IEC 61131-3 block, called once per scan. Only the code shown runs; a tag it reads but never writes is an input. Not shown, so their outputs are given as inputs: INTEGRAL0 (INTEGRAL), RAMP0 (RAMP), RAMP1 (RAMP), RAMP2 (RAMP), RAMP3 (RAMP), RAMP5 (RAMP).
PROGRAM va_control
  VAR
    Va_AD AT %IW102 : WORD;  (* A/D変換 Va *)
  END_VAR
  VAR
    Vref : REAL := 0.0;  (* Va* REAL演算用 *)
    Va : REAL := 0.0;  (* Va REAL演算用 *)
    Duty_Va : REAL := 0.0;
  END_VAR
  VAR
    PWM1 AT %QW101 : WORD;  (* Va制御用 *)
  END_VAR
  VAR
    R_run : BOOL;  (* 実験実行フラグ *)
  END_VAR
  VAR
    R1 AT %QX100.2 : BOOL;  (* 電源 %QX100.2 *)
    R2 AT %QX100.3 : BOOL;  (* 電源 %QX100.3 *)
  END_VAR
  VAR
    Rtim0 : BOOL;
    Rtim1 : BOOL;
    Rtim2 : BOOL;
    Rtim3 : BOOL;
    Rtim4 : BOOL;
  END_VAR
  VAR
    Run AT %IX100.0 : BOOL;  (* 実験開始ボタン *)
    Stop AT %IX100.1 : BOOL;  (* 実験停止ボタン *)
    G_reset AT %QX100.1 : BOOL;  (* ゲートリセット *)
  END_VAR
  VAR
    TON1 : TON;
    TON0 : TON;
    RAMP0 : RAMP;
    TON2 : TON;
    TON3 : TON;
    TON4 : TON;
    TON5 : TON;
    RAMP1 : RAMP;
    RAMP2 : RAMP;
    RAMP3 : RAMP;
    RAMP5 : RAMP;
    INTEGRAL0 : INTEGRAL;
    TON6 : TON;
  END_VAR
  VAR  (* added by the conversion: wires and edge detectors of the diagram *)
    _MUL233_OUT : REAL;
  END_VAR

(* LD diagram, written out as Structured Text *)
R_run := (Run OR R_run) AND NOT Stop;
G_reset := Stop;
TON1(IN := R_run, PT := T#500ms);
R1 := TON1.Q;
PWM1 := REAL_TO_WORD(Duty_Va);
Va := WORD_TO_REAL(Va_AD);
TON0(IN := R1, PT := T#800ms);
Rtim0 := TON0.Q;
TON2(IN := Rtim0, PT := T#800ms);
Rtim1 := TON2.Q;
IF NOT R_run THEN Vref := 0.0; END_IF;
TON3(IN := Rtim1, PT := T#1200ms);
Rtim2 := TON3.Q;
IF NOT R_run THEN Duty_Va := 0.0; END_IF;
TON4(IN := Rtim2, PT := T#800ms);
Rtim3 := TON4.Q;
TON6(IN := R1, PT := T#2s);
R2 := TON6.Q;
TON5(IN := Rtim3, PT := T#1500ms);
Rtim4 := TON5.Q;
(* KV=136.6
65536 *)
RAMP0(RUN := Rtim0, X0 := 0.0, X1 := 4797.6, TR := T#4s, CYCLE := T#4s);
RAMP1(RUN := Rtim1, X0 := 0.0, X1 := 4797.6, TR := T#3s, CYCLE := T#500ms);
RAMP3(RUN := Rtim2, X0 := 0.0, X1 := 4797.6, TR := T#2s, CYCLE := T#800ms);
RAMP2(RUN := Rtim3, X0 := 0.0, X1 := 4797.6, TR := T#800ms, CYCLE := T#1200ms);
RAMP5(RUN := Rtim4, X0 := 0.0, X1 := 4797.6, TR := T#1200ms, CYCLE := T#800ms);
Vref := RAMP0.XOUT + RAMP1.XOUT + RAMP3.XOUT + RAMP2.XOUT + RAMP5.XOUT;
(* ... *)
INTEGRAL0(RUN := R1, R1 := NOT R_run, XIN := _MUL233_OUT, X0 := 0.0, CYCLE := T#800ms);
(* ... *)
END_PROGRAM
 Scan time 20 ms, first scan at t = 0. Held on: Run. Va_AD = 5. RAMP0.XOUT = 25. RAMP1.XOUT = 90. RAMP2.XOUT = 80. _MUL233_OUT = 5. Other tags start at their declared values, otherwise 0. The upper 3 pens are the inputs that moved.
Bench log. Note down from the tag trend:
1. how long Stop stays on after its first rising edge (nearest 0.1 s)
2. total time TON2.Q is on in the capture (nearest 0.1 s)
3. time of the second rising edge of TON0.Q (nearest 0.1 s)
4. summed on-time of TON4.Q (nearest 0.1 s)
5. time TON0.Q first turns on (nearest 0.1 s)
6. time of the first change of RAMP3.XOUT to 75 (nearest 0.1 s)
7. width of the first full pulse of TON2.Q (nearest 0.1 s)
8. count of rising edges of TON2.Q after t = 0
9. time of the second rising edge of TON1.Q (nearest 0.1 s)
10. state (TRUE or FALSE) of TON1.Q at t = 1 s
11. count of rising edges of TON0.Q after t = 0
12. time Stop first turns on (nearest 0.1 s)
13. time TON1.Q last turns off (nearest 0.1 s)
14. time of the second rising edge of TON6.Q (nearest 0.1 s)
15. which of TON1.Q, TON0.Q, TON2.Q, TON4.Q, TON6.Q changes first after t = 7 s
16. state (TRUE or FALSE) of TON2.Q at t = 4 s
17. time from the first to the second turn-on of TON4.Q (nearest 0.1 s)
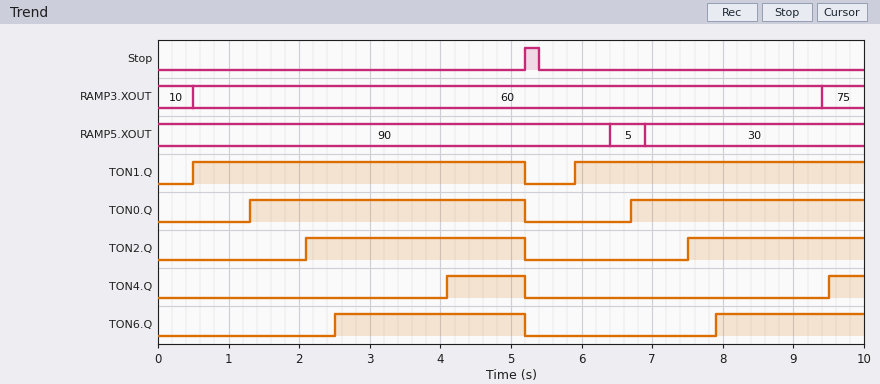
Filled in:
0.2 s
5.6 s
6.7 s
1.6 s
1.3 s
9.4 s
3.1 s
2
5.9 s
TRUE
2
5.2 s
5.2 s
7.9 s
TON2.Q
TRUE
5.4 s
